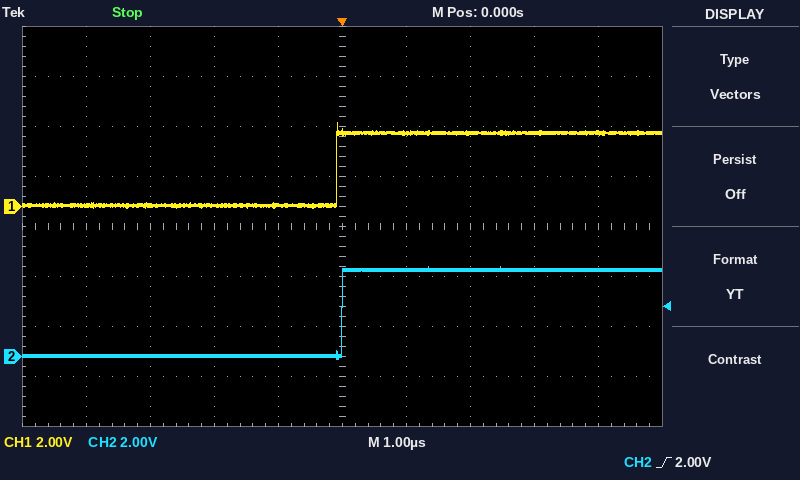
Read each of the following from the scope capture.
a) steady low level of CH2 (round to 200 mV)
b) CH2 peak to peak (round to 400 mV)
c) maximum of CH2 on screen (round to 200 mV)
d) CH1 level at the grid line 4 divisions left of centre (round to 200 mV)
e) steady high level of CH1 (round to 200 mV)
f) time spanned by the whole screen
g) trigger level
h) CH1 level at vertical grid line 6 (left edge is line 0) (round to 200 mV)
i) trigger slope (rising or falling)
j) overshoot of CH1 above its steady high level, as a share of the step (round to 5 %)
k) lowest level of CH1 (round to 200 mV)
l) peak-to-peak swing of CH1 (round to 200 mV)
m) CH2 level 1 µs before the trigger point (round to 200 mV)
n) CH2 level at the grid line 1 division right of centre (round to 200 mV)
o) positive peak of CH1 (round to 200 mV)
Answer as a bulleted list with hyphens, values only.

- 0.0 V
- 3.6 V
- 3.6 V
- 0.0 V
- 3.0 V
- 10 µs
- 2.00 V
- 3.0 V
- rising
- 15 %
- 0.0 V
- 3.4 V
- 0.0 V
- 3.4 V
- 3.4 V
